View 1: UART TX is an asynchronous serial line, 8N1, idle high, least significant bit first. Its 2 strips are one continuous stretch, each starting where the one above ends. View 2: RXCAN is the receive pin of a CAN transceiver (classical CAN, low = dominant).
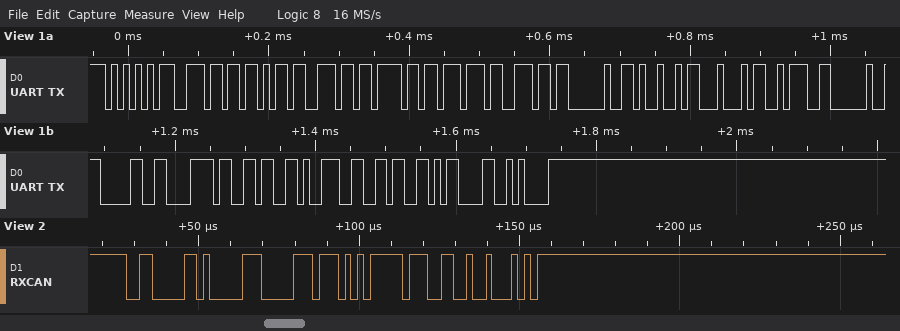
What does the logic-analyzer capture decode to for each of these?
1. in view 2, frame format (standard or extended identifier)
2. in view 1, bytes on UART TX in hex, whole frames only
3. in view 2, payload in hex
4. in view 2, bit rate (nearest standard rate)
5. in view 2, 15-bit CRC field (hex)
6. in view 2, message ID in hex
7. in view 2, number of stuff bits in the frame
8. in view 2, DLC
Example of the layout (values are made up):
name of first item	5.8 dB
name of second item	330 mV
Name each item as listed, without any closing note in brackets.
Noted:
in view 2, frame format	standard
in view 1, bytes on UART TX in hex, whole frames only	0x55 0x6E 0x6B 0x6E 0x6F 0x77 0x6E 0x20 0x49 0x44 0x3A 0x20 0x30 0x78 0x36 0x39 0x36 0x0D 0x0A
in view 2, payload in hex	06 EA FF
in view 2, bit rate	500 kbit/s
in view 2, 15-bit CRC field	0x1922
in view 2, message ID in hex	0x305
in view 2, number of stuff bits in the frame	4
in view 2, DLC	3
